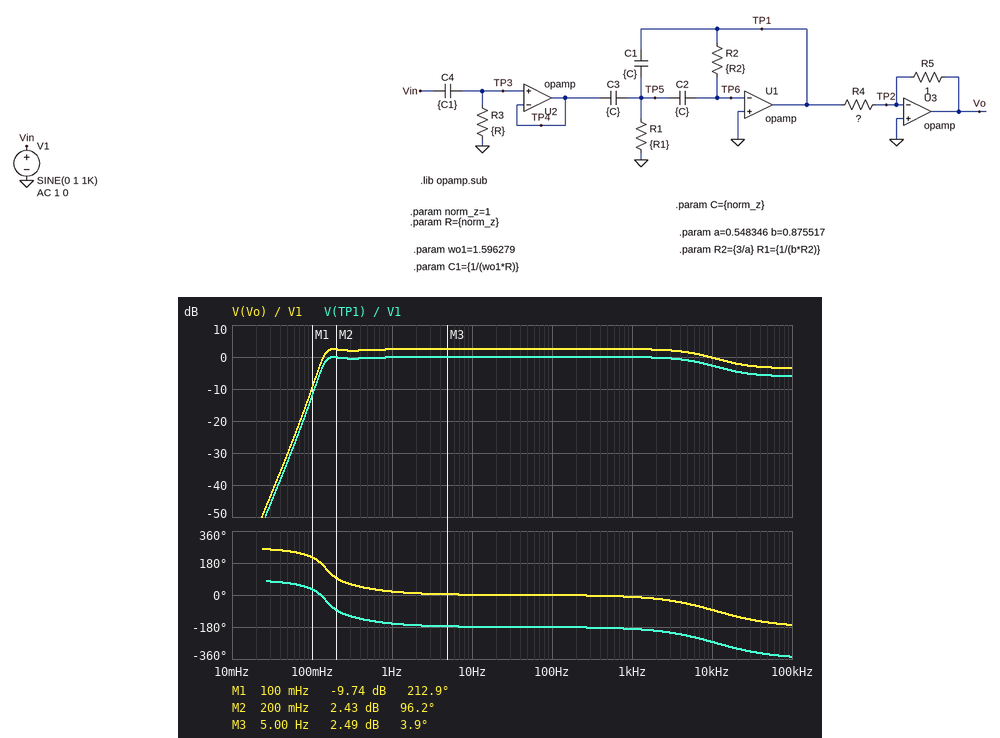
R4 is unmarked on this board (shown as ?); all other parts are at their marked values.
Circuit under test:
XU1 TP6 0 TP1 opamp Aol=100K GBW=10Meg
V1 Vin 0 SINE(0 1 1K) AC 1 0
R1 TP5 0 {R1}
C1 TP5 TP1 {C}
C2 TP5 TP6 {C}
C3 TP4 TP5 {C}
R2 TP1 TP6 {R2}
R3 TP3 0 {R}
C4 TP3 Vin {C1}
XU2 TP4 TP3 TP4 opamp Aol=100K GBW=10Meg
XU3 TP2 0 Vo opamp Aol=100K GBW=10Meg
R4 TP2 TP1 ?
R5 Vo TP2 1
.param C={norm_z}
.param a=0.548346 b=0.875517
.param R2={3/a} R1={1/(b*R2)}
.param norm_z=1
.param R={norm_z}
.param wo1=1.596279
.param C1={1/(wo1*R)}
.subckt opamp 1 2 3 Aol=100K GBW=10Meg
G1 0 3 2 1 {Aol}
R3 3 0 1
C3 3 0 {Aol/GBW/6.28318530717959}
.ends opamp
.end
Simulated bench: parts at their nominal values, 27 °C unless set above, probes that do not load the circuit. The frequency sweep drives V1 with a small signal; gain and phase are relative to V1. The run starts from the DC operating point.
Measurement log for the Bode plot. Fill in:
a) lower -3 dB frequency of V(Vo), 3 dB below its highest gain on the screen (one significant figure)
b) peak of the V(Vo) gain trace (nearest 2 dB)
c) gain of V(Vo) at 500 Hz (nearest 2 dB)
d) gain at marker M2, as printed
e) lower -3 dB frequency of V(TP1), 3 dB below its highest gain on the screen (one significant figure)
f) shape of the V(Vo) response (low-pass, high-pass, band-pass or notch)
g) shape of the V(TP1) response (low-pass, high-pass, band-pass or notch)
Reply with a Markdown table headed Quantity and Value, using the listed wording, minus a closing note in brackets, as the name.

| Quantity | Value |
|---|---|
| lower -3 dB frequency of V(Vo), 3 dB below its highest gain on the screen | 100 mHz |
| peak of the V(Vo) gain trace | 2 dB |
| gain of V(Vo) at 500 Hz | 2 dB |
| gain at marker M2, as printed | 2.43 dB |
| lower -3 dB frequency of V(TP1), 3 dB below its highest gain on the screen | 100 mHz |
| shape of the V(Vo) response | high-pass |
| shape of the V(TP1) response | high-pass |
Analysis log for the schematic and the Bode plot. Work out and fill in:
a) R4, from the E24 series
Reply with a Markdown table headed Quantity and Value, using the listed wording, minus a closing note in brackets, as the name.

| Quantity | Value |
|---|---|
| R4, from the E24 series | 0.75 Ω |
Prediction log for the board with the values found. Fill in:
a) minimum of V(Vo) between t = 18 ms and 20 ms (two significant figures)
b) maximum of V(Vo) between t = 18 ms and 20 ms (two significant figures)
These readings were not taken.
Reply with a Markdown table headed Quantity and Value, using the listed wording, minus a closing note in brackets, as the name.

| Quantity | Value |
|---|---|
| minimum of V(Vo) between t = 18 ms and 20 ms | -1.3 V |
| maximum of V(Vo) between t = 18 ms and 20 ms | 1.3 V |
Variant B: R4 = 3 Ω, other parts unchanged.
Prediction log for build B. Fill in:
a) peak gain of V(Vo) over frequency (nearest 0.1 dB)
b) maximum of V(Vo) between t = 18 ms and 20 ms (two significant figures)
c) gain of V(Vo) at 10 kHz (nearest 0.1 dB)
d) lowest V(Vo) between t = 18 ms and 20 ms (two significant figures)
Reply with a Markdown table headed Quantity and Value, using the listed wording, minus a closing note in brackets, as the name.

| Quantity | Value |
|---|---|
| peak gain of V(Vo) over frequency | -9.5 dB |
| maximum of V(Vo) between t = 18 ms and 20 ms | 330 mV |
| gain of V(Vo) at 10 kHz | -12.2 dB |
| lowest V(Vo) between t = 18 ms and 20 ms | -330 mV |
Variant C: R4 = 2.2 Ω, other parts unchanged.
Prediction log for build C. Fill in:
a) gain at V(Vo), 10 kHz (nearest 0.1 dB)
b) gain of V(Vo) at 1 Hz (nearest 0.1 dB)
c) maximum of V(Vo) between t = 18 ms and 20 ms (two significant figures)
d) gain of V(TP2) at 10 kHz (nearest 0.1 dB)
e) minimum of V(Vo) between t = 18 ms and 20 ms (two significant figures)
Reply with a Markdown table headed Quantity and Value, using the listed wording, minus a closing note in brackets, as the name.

| Quantity | Value |
|---|---|
| gain at V(Vo), 10 kHz | -9.5 dB |
| gain of V(Vo) at 1 Hz | -7.0 dB |
| maximum of V(Vo) between t = 18 ms and 20 ms | 450 mV |
| gain of V(TP2) at 10 kHz | -69.5 dB |
| minimum of V(Vo) between t = 18 ms and 20 ms | -450 mV |
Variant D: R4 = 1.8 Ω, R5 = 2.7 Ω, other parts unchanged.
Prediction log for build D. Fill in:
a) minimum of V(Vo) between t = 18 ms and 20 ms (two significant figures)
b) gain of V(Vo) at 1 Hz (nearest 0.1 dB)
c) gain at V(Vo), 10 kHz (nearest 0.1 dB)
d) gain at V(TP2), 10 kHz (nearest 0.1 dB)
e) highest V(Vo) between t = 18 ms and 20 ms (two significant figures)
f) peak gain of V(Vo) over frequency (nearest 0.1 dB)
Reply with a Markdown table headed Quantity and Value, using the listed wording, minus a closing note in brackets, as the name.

| Quantity | Value |
|---|---|
| minimum of V(Vo) between t = 18 ms and 20 ms | -1.5 V |
| gain of V(Vo) at 1 Hz | 3.4 dB |
| gain at V(Vo), 10 kHz | 0.8 dB |
| gain at V(TP2), 10 kHz | -59.2 dB |
| highest V(Vo) between t = 18 ms and 20 ms | 1.5 V |
| peak gain of V(Vo) over frequency | 3.5 dB |
